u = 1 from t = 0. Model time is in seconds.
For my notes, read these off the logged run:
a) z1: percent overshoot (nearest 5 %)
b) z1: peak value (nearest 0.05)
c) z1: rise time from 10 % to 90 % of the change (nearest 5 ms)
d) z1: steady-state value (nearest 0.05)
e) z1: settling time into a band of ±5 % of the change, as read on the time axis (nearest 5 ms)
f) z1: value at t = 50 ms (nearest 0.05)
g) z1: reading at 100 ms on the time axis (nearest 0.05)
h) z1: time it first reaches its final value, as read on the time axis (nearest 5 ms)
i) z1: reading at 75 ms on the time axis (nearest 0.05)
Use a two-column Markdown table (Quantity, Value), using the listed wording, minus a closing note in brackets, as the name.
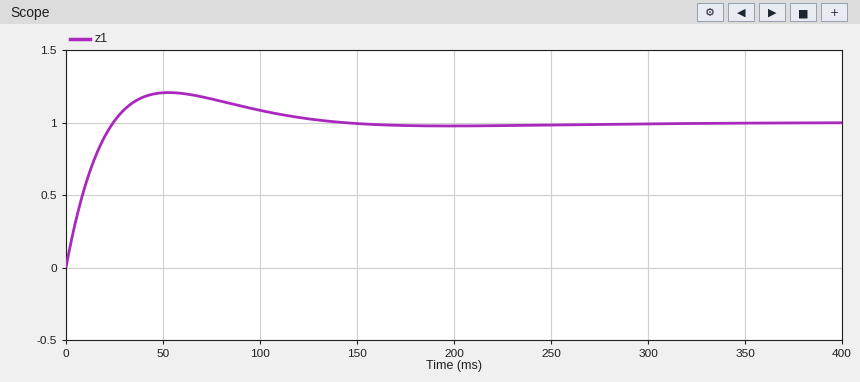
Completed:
| Quantity | Value |
|---|---|
| z1: percent overshoot | 20 % |
| z1: peak value | 1.20 |
| z1: rise time from 10 % to 90 % of the change | 20 ms |
| z1: steady-state value | 1.00 |
| z1: settling time into a band of ±5 % of the change, as read on the time axis | 115 ms |
| z1: value at t = 50 ms | 1.20 |
| z1: reading at 100 ms on the time axis | 1.10 |
| z1: time it first reaches its final value, as read on the time axis | 25 ms |
| z1: reading at 75 ms on the time axis | 1.15 |
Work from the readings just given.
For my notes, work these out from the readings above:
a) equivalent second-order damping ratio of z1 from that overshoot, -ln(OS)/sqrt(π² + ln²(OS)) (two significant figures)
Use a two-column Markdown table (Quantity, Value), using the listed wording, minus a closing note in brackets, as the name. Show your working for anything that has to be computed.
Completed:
| Quantity | Value |
|---|---|
| equivalent second-order damping ratio of z1 from that overshoot, -ln(OS)/sqrt(π² + ln²(OS)) | ln(0.2) = -1.609; 1.609 / sqrt(9.870 + 2.590) = 0.46 |
